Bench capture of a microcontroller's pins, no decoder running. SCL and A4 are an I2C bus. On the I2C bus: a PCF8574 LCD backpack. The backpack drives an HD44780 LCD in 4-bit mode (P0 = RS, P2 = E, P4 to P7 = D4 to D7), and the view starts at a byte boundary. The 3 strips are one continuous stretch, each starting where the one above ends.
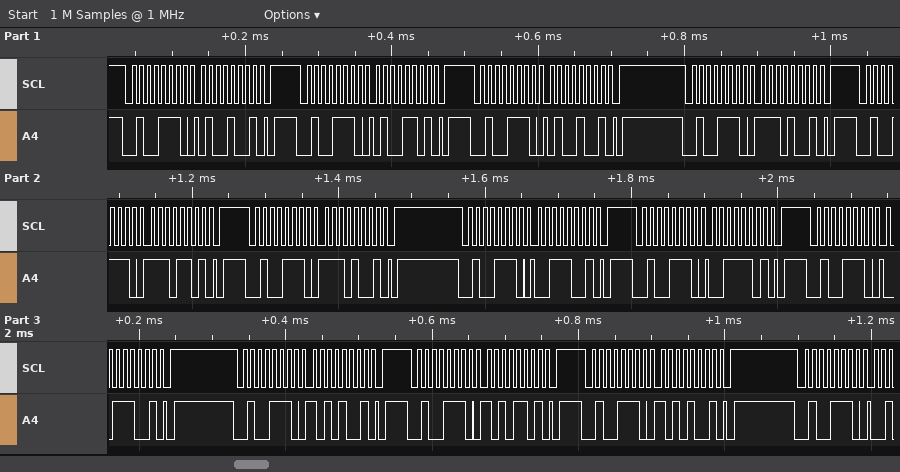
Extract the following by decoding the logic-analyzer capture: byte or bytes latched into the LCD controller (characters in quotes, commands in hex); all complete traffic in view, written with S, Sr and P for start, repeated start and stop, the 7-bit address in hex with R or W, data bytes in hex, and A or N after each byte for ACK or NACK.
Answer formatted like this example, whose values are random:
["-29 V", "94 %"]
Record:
["'N' ':'", "S 27W A 49 A P S 27W A 4D A P S 27W A 49 A P S 27W A E9 A P S 27W A ED A P S 27W A E9 A P S 27W A 39 A P S 27W A 3D A P S 27W A 39 A P S 27W A A9 A P S 27W A AD A P S 27W A A9 A P S 27W A"]
